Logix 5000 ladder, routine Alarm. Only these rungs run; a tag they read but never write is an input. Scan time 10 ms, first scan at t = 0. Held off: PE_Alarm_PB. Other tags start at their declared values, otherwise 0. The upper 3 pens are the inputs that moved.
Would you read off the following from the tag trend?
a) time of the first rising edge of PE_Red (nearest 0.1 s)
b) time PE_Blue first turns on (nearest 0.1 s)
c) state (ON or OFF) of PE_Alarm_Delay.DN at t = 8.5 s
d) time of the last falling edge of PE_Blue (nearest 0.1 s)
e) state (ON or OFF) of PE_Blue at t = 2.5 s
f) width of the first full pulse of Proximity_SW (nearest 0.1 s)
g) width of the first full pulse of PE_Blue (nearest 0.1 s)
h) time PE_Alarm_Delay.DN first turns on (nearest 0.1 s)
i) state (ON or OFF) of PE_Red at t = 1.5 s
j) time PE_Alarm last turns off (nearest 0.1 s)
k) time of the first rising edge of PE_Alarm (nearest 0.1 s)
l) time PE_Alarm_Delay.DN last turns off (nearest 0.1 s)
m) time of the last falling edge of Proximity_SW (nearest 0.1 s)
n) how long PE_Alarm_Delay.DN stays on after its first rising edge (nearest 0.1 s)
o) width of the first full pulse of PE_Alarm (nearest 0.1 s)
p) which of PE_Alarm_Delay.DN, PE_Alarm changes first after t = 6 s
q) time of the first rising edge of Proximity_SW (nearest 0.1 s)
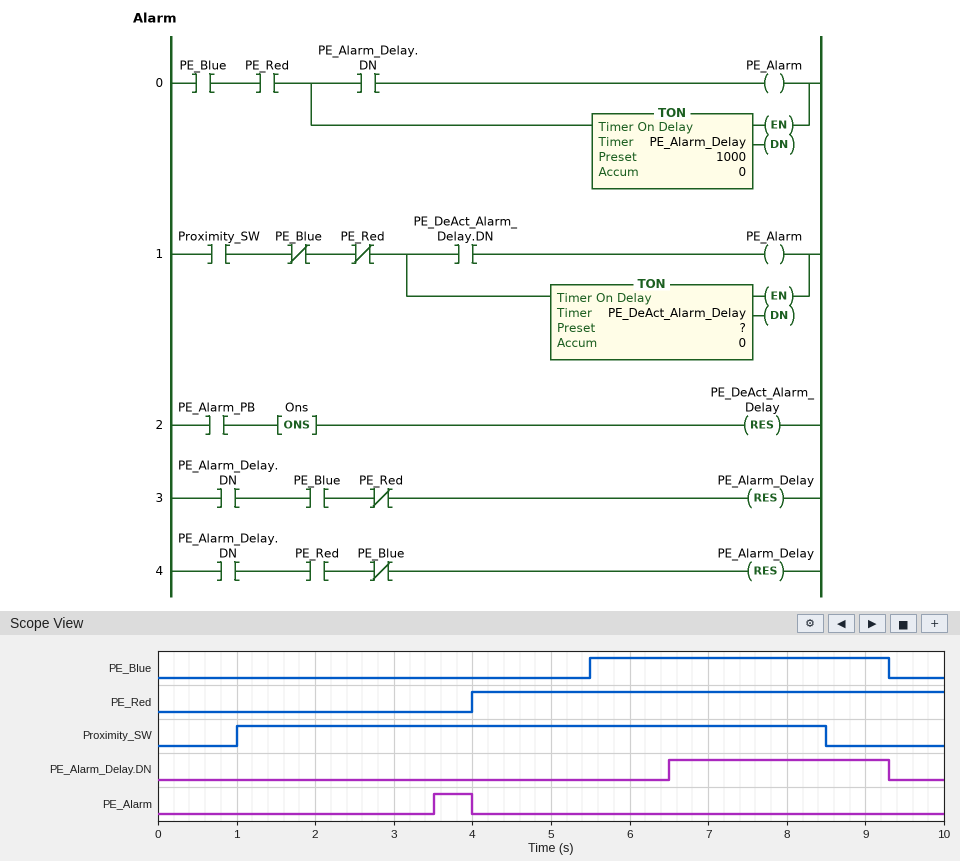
4.0 s
5.5 s
ON
9.3 s
OFF
7.5 s
3.8 s
6.5 s
OFF
4.0 s
3.5 s
9.3 s
8.5 s
2.8 s
0.5 s
PE_Alarm_Delay.DN
1.0 s
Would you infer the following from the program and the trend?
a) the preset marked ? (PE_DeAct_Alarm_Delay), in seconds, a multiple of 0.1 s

2.5 s
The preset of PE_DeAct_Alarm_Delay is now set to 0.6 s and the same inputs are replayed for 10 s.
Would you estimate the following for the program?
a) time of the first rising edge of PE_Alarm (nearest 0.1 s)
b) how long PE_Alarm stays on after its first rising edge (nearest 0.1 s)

1.6 s
2.4 s
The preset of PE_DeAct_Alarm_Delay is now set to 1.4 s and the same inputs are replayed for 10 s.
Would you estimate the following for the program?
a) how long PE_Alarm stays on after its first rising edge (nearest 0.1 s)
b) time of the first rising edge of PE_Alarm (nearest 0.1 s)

1.6 s
2.4 s
